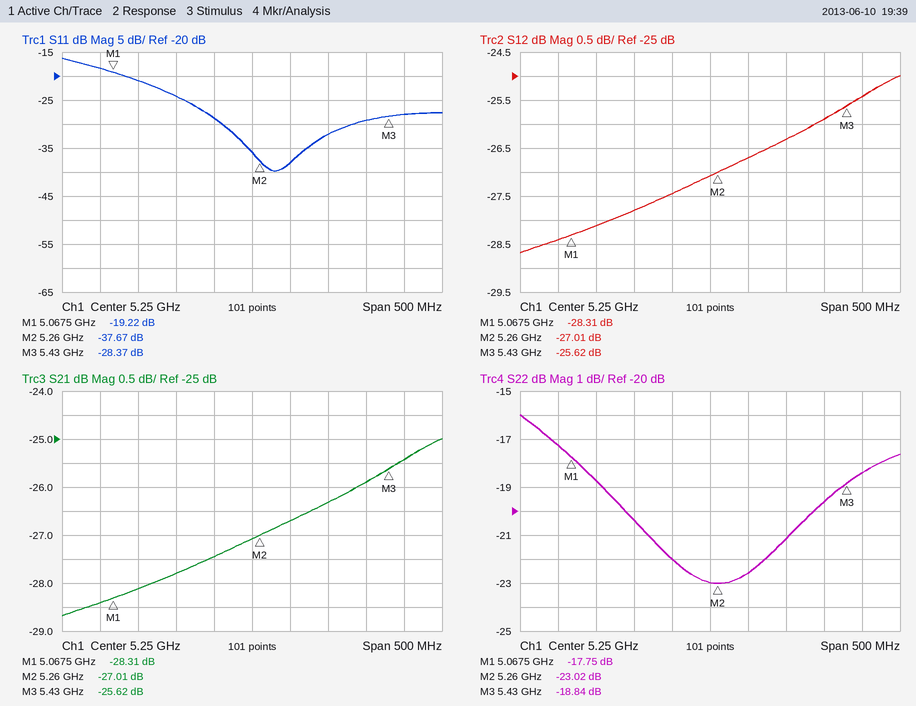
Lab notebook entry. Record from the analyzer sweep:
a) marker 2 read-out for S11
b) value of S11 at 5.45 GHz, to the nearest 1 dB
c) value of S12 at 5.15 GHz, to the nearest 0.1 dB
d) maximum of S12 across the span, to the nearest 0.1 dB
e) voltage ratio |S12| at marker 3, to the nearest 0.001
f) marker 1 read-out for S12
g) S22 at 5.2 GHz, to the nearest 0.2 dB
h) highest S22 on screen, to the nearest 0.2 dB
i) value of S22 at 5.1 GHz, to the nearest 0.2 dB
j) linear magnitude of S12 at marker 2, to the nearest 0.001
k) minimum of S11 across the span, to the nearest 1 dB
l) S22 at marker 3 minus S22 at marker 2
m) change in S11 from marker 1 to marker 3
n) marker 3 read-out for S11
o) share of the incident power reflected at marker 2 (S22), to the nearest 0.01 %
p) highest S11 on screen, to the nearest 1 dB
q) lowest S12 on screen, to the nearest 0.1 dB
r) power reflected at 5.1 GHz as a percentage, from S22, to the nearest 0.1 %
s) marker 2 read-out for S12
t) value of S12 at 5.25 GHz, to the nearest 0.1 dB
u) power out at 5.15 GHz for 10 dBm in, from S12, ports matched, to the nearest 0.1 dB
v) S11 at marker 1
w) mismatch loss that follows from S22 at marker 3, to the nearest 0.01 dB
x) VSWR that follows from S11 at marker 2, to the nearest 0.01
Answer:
-37.67 dB
-28 dB
-27.8 dB
-25.0 dB
0.052
-28.31 dB
-22.0 dB
-16.0 dB
-18.8 dB
0.045
-40 dB
4.18 dB
-9.15 dB
-28.37 dB
0.50 %
-16 dB
-28.7 dB
1.3 %
-27.01 dB
-27.1 dB
-17.8 dBm
-19.22 dB
0.06 dB
1.03
